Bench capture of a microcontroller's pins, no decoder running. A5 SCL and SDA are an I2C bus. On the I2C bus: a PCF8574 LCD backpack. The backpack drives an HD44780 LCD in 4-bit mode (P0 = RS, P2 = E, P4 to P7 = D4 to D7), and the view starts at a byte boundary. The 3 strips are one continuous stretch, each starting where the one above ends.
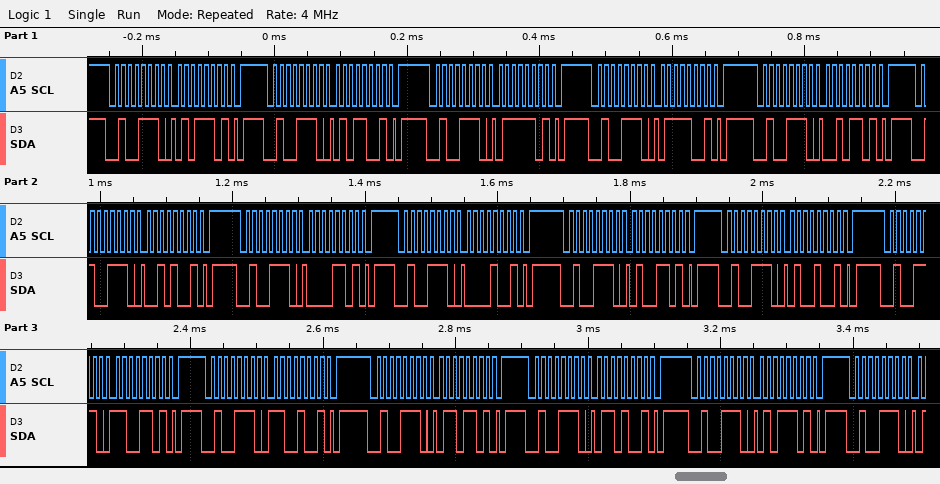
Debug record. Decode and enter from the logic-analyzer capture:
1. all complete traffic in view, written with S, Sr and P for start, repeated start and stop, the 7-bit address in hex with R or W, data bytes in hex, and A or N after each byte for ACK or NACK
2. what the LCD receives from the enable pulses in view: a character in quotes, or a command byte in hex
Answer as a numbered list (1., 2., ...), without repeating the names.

1. S 27W A 5D A P S 27W A 59 A P S 27W A 7D A P S 27W A 79 A P S 27W A 2D A P S 27W A 29 A P S 27W A 0D A P S 27W A 09 A P S 27W A 4D A P S 27W A 49 A P S 27W A CD A P S 27W A C9 A P S 27W A 6D A P S 27W A 69 A P S 27W A 5D A P S 27W A
2. 'W' ' ' 'L'
